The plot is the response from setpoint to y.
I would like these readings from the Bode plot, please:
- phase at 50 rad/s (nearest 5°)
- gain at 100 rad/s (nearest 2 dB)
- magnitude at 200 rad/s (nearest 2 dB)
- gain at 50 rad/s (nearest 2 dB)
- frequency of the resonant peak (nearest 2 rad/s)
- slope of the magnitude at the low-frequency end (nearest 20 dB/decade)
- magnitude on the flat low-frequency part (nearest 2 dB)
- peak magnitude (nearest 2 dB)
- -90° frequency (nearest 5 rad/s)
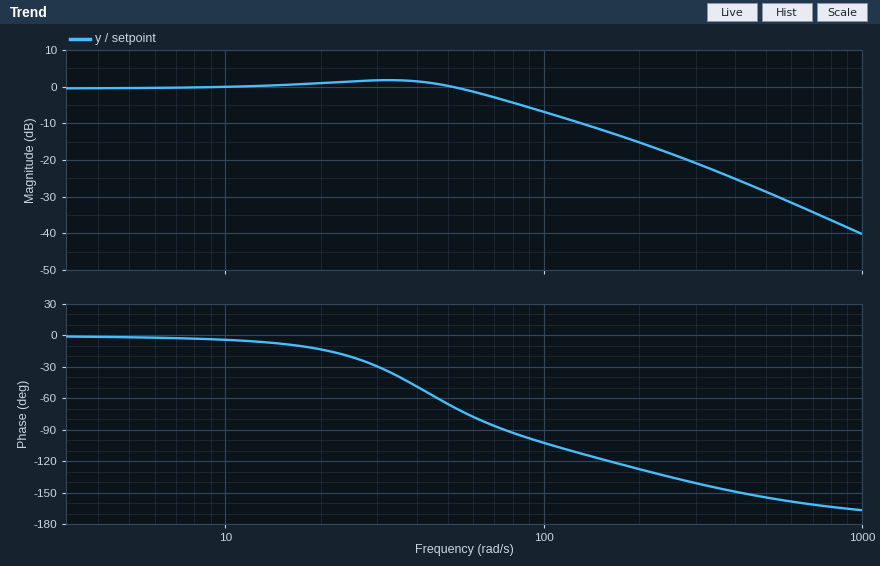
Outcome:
-65°
-6 dB
-16 dB
0 dB
32 rad/s
0 dB/decade
0 dB
2 dB
75 rad/s
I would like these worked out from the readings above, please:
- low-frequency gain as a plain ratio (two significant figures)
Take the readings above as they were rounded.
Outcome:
1.0
